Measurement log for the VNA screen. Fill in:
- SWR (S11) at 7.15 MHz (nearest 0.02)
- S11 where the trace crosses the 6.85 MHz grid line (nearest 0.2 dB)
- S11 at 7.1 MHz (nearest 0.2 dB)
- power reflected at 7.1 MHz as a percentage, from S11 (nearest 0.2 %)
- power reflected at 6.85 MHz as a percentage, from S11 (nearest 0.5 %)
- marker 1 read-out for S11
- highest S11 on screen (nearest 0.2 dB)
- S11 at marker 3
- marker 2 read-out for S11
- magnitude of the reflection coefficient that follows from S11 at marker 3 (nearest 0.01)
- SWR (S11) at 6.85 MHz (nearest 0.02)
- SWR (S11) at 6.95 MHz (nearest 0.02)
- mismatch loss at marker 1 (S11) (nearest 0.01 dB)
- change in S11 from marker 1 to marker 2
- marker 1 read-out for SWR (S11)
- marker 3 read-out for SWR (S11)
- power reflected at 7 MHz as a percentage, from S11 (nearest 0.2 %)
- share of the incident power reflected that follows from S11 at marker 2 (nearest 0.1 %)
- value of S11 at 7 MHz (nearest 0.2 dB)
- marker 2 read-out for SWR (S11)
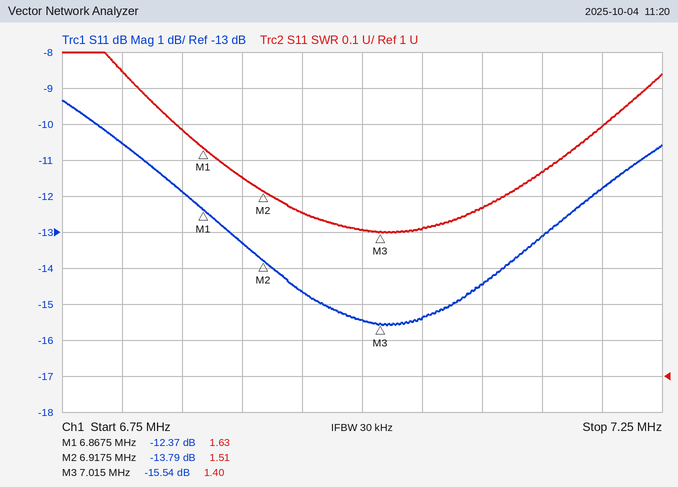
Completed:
1.56
-11.8 dB
-14.4 dB
3.6 %
6.5 %
-12.37 dB
-9.4 dB
-15.54 dB
-13.79 dB
0.17
1.68
1.46
0.26 dB
-1.42 dB
1.63
1.40
2.8 %
4.2 %
-15.4 dB
1.51
